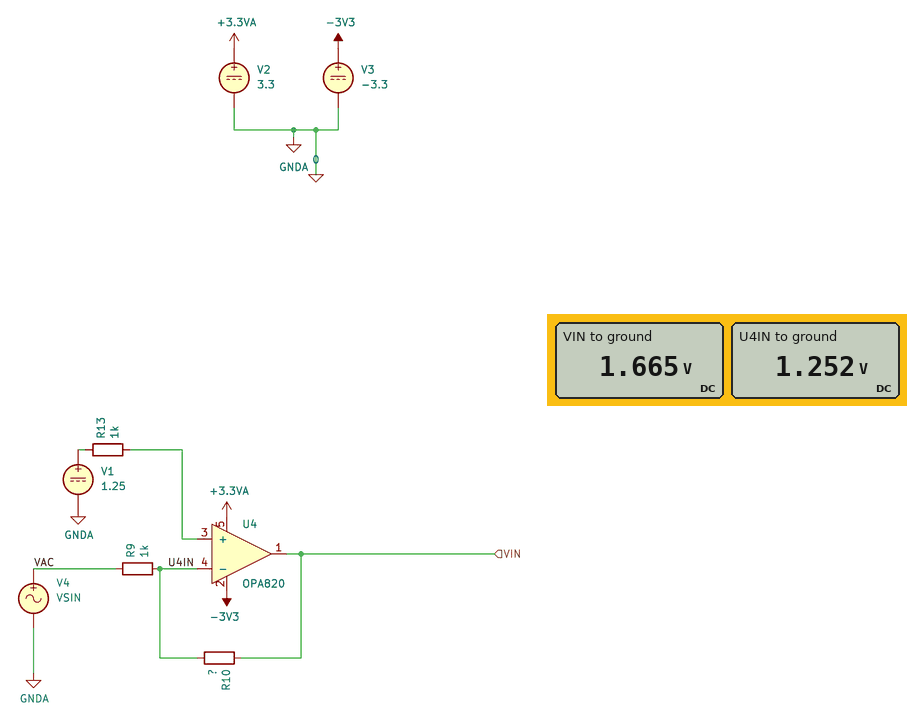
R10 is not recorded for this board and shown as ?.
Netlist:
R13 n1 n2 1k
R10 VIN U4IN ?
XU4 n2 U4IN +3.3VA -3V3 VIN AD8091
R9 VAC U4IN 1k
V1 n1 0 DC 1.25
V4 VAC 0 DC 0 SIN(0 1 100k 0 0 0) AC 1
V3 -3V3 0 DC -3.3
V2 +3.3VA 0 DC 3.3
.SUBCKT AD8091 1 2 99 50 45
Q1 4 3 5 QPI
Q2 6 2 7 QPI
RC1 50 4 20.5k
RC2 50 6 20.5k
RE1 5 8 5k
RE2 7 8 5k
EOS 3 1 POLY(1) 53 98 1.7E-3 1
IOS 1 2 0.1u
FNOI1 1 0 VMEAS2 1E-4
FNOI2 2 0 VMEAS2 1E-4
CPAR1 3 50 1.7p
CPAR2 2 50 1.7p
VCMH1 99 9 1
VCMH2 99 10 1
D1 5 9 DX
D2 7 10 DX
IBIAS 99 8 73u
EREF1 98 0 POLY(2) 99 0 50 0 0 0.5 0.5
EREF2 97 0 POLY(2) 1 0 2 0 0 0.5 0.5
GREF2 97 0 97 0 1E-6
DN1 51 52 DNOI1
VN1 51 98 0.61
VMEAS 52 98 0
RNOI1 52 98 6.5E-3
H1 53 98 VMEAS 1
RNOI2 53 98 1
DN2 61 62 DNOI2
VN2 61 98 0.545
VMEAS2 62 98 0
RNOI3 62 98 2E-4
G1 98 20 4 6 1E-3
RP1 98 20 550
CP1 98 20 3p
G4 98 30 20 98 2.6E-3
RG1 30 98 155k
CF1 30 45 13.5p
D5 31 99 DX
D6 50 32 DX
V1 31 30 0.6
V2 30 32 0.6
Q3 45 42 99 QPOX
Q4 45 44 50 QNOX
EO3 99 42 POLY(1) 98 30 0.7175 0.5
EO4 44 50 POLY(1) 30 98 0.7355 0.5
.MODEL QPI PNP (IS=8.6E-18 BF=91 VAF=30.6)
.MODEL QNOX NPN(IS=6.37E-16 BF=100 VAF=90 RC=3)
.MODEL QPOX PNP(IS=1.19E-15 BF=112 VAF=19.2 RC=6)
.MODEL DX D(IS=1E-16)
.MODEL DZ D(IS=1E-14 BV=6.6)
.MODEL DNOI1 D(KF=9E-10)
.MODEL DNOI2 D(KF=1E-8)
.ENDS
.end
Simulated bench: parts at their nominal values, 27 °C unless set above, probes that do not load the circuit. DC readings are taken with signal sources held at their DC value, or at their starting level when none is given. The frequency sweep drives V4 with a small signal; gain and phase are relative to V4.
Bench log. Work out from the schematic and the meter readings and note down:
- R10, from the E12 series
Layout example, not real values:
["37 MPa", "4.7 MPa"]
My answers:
["330 Ω"]
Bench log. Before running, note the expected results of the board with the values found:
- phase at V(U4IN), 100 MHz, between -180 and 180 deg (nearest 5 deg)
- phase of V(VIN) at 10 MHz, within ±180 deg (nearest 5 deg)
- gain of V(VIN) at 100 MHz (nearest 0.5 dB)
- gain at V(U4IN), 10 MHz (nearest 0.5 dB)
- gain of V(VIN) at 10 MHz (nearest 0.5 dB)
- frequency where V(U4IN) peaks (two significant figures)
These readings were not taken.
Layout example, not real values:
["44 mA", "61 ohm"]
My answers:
["-5 deg", "165 deg", "-16.5 dB", "-24.5 dB", "-9.5 dB", "71 MHz"]
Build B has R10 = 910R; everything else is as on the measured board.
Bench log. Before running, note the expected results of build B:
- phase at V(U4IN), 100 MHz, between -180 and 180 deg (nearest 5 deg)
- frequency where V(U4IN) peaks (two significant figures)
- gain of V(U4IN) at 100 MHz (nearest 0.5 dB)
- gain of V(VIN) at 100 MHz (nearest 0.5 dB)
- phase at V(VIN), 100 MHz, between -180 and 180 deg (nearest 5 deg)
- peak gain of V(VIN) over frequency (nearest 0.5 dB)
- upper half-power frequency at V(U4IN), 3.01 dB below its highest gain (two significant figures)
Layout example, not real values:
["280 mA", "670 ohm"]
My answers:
["-25 deg", "56 MHz", "-5.5 dB", "-13.0 dB", "10 deg", "-1.0 dB", "130 MHz"]
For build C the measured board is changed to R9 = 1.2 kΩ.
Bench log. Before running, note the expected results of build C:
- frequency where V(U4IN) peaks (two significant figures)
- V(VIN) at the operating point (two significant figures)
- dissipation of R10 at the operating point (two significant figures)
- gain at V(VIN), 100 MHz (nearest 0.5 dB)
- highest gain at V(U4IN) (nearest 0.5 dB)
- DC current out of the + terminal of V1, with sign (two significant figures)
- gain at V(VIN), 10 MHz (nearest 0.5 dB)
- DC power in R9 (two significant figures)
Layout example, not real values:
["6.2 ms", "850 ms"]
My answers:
["72 MHz", "1.6 V", "360 µW", "-17.5 dB", "-9.5 dB", "-250 nA", "-11.0 dB", "1.3 mW"]
